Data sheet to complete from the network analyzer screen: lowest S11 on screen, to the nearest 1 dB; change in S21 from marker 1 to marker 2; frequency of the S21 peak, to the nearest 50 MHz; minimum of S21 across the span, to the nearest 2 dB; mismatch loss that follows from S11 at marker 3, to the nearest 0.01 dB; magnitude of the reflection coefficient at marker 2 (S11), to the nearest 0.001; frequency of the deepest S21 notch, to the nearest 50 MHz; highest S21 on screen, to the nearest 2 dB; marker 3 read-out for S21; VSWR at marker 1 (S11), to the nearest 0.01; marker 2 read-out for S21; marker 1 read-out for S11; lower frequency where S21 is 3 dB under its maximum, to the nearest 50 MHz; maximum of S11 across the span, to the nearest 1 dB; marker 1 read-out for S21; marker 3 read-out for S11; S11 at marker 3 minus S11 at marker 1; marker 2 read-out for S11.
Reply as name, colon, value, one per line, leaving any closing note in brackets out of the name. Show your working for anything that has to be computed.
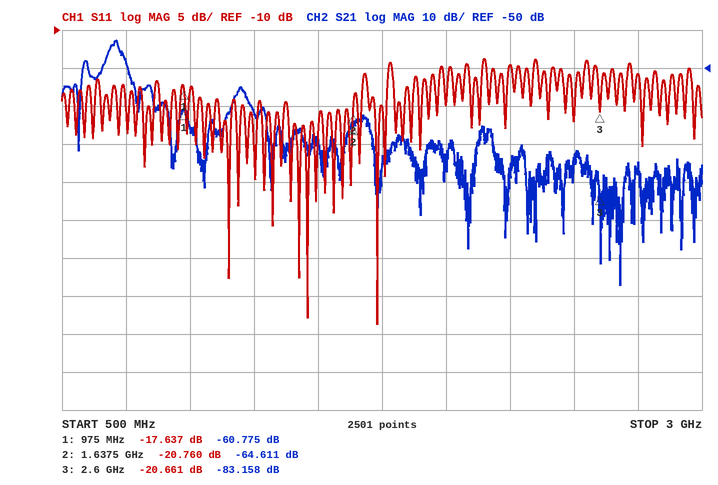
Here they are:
lowest S11 on screen, to the nearest 1 dB: -49 dB
change in S21 from marker 1 to marker 2: -64.611 − (-60.775) = -3.836 dB
frequency of the S21 peak, to the nearest 50 MHz: 700 MHz
minimum of S21 across the span, to the nearest 2 dB: -108 dB
mismatch loss that follows from S11 at marker 3, to the nearest 0.01 dB: −10 log10(1 − 10^(-20.661/10)) ≈ 0.04 dB
magnitude of the reflection coefficient at marker 2 (S11), to the nearest 0.001: 10^(-20.76/20) ≈ 0.092
frequency of the deepest S21 notch, to the nearest 50 MHz: 2.70 GHz
highest S21 on screen, to the nearest 2 dB: -42 dB
marker 3 read-out for S21: -83.158 dB
VSWR at marker 1 (S11), to the nearest 0.01: (1 + 0.1313)/(1 − 0.1313) ≈ 1.30
marker 2 read-out for S21: -64.611 dB
marker 1 read-out for S11: -17.637 dB
lower frequency where S21 is 3 dB under its maximum, to the nearest 50 MHz: 700 MHz
maximum of S11 across the span, to the nearest 1 dB: -14 dB
marker 1 read-out for S21: -60.775 dB
marker 3 read-out for S11: -20.661 dB
S11 at marker 3 minus S11 at marker 1: -20.661 − (-17.637) = -3.024 dB
marker 2 read-out for S11: -20.760 dB
